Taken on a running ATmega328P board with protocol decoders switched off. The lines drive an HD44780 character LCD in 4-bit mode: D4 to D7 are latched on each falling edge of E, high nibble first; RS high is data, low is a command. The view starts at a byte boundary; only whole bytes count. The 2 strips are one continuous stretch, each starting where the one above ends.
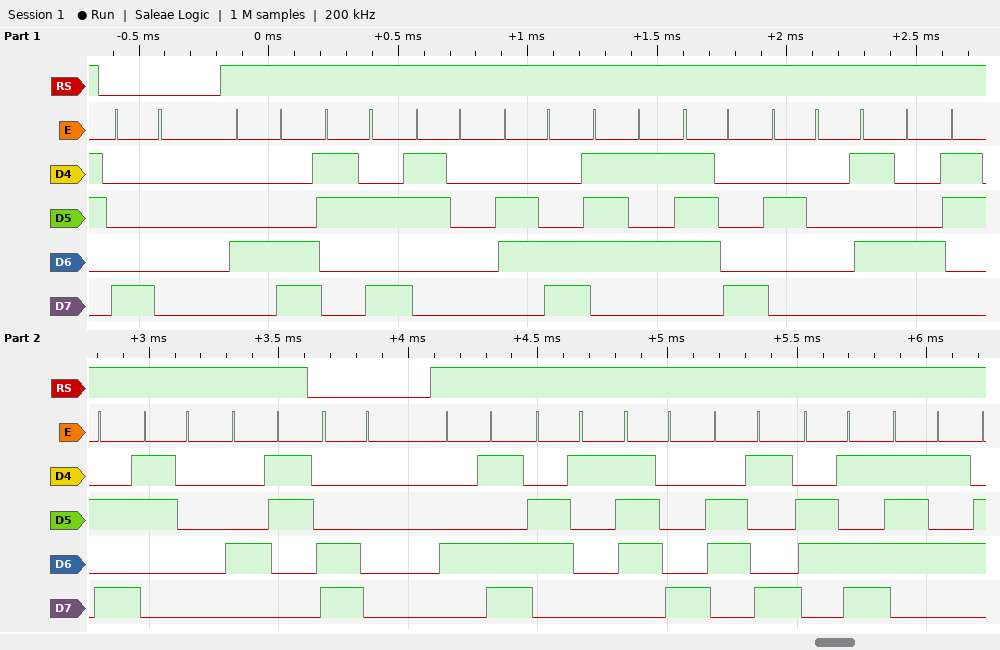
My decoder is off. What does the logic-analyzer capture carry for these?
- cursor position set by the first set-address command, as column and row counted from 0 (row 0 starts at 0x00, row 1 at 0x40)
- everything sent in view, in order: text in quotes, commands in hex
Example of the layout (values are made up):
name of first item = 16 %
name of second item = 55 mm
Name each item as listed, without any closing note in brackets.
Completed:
cursor position set by the first set-address command, as column and row counted from 0 = column 0, row 0
everything sent in view, in order: text in quotes, commands in hex = 0x80 "L:0lux T:0C" 0xC0 "Maximu"
